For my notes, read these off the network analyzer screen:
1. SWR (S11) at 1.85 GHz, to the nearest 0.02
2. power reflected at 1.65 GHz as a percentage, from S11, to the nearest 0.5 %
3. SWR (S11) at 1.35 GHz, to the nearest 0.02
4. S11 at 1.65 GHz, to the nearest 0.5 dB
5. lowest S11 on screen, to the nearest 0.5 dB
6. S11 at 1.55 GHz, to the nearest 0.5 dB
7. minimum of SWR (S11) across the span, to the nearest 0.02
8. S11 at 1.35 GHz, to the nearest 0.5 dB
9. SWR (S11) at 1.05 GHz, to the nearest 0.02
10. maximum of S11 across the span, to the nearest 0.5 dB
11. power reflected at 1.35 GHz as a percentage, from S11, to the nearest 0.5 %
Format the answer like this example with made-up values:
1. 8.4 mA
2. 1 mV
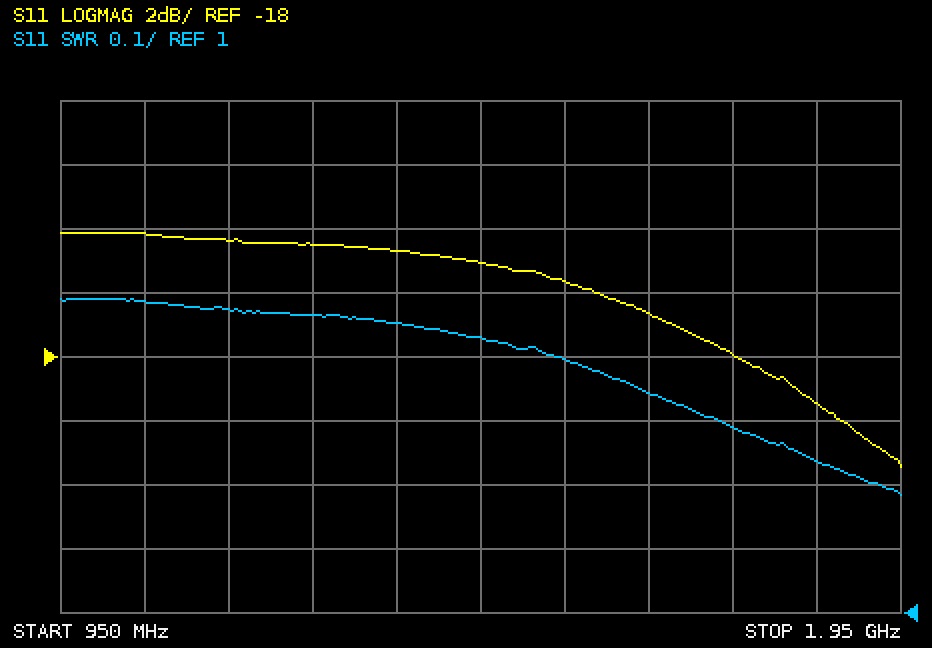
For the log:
1. 1.24
2. 2.0 %
3. 1.46
4. -16.5 dB
5. -21.5 dB
6. -15.5 dB
7. 1.18
8. -14.5 dB
9. 1.48
10. -14.0 dB
11. 3.5 %
